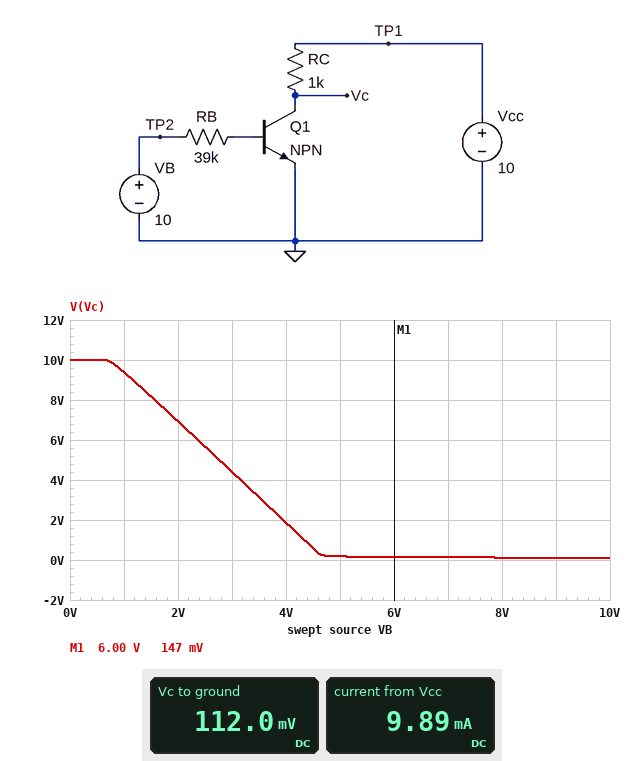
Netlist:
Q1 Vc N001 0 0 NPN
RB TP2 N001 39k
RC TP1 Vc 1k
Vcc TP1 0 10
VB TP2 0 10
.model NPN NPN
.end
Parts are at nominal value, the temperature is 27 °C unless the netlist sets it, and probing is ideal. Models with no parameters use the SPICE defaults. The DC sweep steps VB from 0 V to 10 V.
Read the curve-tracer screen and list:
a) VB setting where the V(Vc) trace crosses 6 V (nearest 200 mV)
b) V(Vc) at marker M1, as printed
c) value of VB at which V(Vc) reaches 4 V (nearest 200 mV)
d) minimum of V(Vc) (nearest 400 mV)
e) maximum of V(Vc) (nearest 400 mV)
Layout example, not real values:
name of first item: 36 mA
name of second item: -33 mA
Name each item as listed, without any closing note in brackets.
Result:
VB setting where the V(Vc) trace crosses 6 V: 2.4 V
V(Vc) at marker M1, as printed: 147 mV
value of VB at which V(Vc) reaches 4 V: 3.2 V
minimum of V(Vc): 0 V
maximum of V(Vc): 10.0 V
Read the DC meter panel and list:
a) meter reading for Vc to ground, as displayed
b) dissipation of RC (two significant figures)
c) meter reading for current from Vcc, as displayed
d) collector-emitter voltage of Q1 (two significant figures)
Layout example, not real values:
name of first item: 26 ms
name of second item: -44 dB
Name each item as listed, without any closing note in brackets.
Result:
meter reading for Vc to ground, as displayed: 112.0 mV
dissipation of RC: 98 mW
meter reading for current from Vcc, as displayed: 9.89 mA
collector-emitter voltage of Q1: 110 mV
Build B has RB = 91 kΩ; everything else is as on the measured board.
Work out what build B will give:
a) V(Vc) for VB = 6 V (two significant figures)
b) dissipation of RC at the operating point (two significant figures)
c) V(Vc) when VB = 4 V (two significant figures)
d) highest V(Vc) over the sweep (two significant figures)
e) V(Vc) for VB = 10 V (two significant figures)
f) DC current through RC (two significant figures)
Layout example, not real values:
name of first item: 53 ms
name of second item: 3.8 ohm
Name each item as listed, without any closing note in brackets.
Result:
V(Vc) for VB = 6 V: 4.3 V
dissipation of RC at the operating point: 96 mW
V(Vc) when VB = 4 V: 6.5 V
highest V(Vc) over the sweep: 10 V
V(Vc) for VB = 10 V: 210 mV
DC current through RC: 9.8 mA
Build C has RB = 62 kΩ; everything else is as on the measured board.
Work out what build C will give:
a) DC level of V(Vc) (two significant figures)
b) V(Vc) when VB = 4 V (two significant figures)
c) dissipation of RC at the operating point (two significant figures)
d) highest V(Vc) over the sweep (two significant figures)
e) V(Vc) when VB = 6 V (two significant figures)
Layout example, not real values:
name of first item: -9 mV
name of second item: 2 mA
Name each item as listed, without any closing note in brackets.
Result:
DC level of V(Vc): 140 mV
V(Vc) when VB = 4 V: 4.9 V
dissipation of RC at the operating point: 97 mW
highest V(Vc) over the sweep: 10 V
V(Vc) when VB = 6 V: 1.7 V
